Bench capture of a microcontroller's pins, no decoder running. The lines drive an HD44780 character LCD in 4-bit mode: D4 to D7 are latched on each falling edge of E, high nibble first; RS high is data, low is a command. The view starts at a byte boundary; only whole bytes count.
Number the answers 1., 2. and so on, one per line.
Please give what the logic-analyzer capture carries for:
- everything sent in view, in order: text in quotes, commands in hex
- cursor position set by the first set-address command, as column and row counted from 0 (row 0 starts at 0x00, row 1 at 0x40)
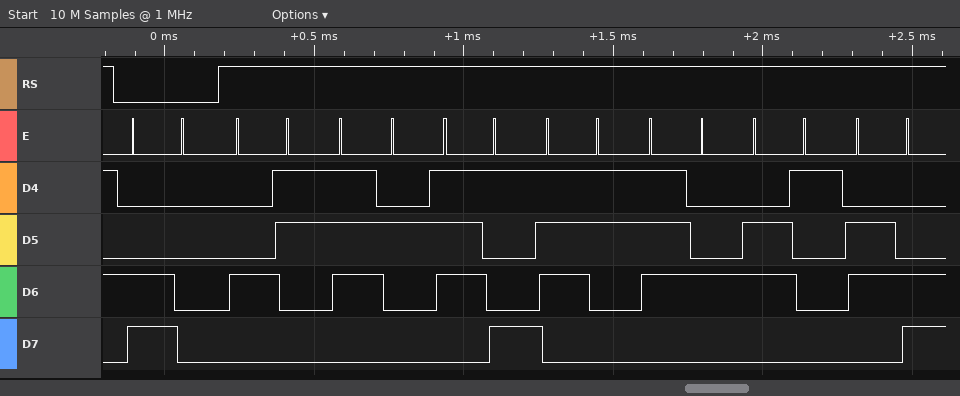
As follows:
1. 0xC0 "Crystal"
2. column 0, row 1
